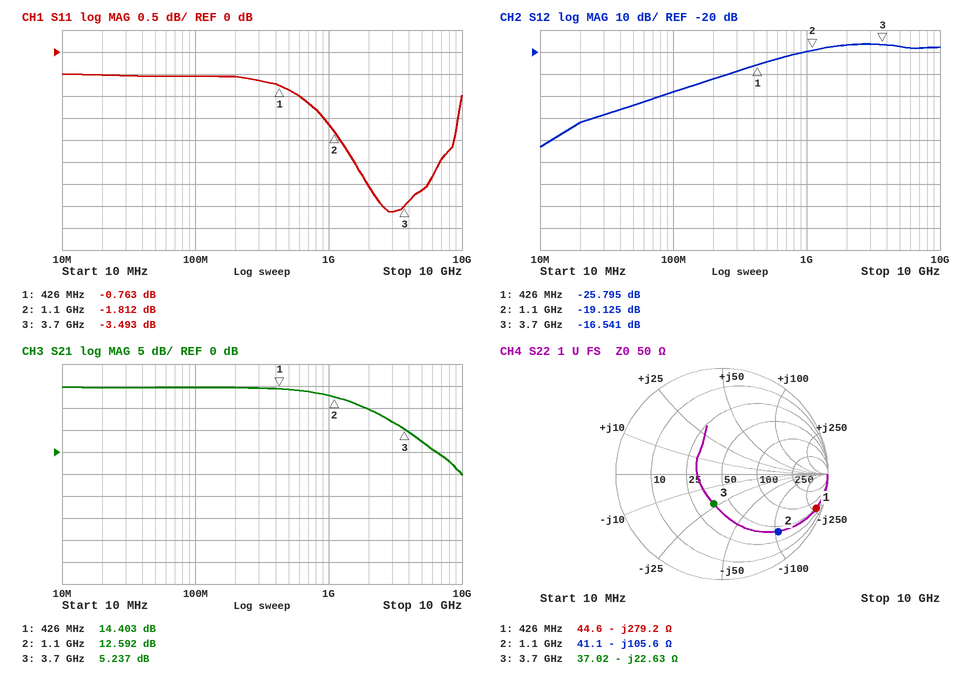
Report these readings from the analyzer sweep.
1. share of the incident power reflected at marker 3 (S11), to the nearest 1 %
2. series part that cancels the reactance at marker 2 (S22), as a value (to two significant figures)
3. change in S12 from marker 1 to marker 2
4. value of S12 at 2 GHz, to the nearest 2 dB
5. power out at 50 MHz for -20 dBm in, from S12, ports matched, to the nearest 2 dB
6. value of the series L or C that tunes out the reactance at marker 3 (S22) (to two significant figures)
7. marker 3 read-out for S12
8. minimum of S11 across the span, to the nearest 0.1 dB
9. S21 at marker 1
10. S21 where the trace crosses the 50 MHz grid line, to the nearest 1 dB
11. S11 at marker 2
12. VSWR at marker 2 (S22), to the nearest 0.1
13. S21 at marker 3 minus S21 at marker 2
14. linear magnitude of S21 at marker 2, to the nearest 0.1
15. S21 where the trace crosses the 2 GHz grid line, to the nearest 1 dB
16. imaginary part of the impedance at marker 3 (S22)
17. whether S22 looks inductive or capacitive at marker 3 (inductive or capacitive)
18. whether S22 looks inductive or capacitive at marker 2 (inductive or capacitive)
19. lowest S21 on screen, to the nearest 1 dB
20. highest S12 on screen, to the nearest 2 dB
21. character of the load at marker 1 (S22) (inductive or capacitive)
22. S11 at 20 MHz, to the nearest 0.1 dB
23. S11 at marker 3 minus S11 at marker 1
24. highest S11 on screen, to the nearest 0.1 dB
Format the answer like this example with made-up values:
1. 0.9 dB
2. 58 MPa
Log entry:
1. 45 %
2. 15 nH
3. 6.670 dB
4. -16 dB
5. -64 dBm
6. 970 pH
7. -16.541 dB
8. -3.6 dB
9. 14.403 dB
10. 15 dB
11. -1.812 dB
12. 7.3
13. -7.355 dB
14. 4.3
15. 10 dB
16. -22.63 Ω
17. capacitive
18. capacitive
19. -5 dB
20. -16 dB
21. capacitive
22. -0.5 dB
23. -2.730 dB
24. -0.5 dB
